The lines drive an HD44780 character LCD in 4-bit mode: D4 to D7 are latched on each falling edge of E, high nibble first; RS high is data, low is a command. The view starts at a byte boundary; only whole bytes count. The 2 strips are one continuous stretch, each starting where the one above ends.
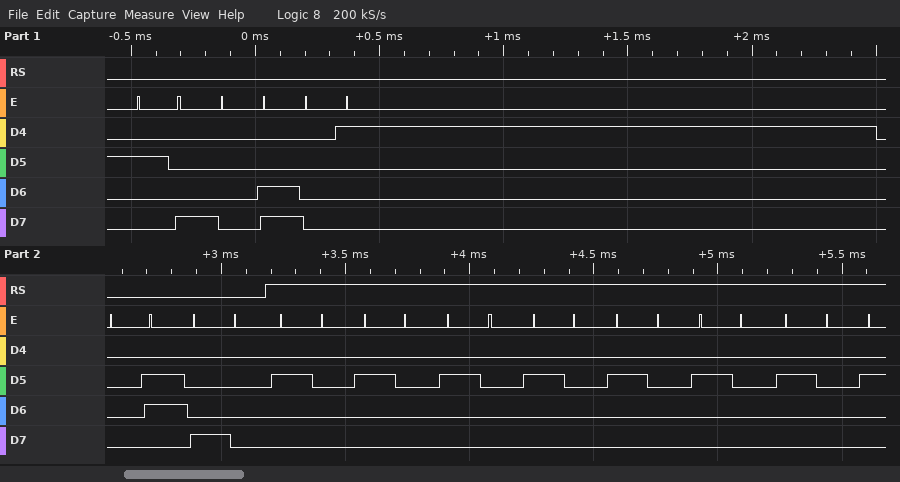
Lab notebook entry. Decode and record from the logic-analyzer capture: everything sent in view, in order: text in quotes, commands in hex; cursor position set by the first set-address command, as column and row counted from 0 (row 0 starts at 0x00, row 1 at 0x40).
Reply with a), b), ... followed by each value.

a) 0x28 0x0C 0x01 0x06 0x80 "       "
b) column 0, row 0
